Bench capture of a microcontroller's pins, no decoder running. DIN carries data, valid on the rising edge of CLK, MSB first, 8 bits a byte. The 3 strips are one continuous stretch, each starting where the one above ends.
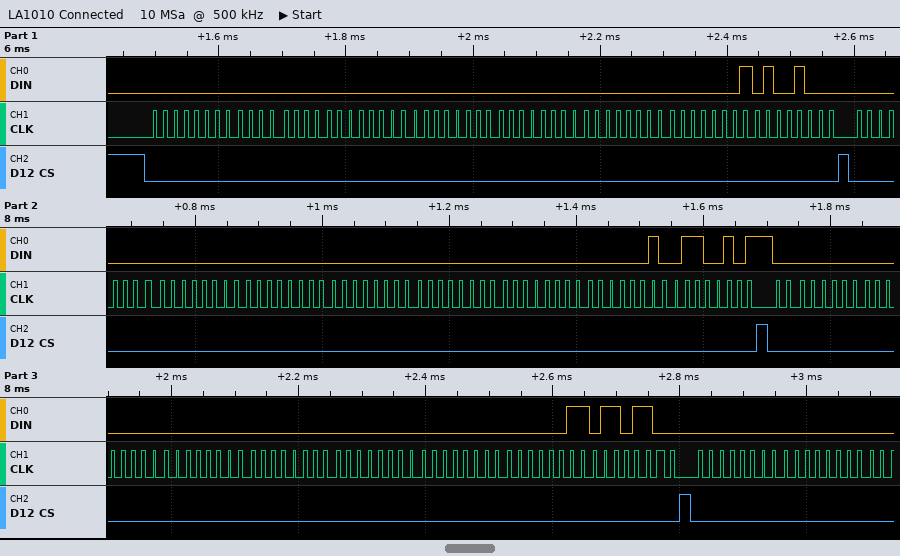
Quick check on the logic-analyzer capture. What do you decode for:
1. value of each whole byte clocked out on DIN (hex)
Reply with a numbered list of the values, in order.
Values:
1. 0x00 0x00 0x00 0x00 0x00 0x00 0x01 0x48 0x00 0x00 0x00 0x00 0x00 0x00 0x02 0x65 0x00 0x00 0x00 0x00 0x00 0x00 0x03 0x6C 0x00 0x00
